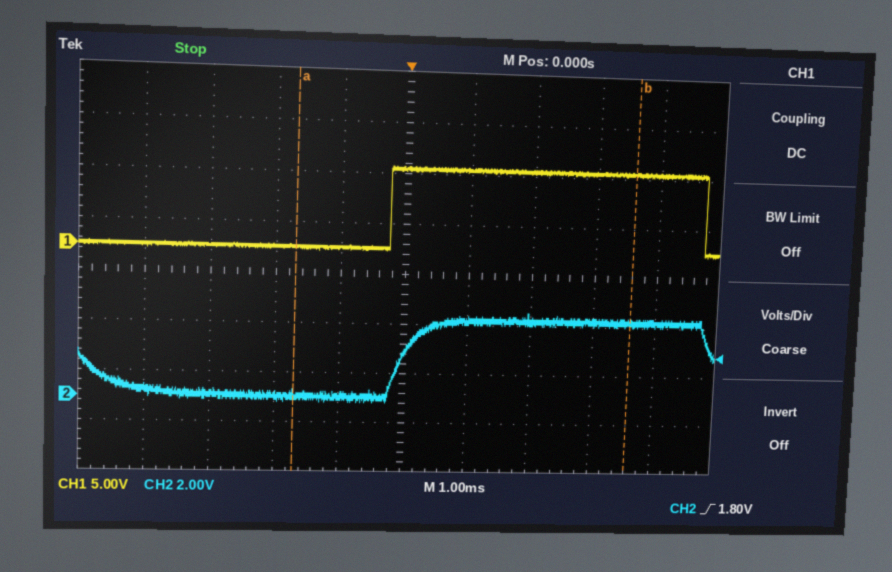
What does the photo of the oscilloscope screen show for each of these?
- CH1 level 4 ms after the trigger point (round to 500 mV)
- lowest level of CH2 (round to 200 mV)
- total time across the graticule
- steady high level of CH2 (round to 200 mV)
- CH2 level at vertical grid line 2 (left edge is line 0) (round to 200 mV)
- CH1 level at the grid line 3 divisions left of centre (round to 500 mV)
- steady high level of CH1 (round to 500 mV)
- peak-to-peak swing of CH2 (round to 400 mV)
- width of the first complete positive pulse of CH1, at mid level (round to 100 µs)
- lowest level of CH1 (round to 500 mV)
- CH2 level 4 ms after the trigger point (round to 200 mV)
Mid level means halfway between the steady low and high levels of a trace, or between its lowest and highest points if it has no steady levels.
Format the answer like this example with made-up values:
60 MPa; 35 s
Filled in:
8.0 V; -200 mV; 10 ms; 3.2 V; 200 mV; 0.0 V; 8.0 V; 3.6 V; 5.0 ms; 0.0 V; 3.2 V
